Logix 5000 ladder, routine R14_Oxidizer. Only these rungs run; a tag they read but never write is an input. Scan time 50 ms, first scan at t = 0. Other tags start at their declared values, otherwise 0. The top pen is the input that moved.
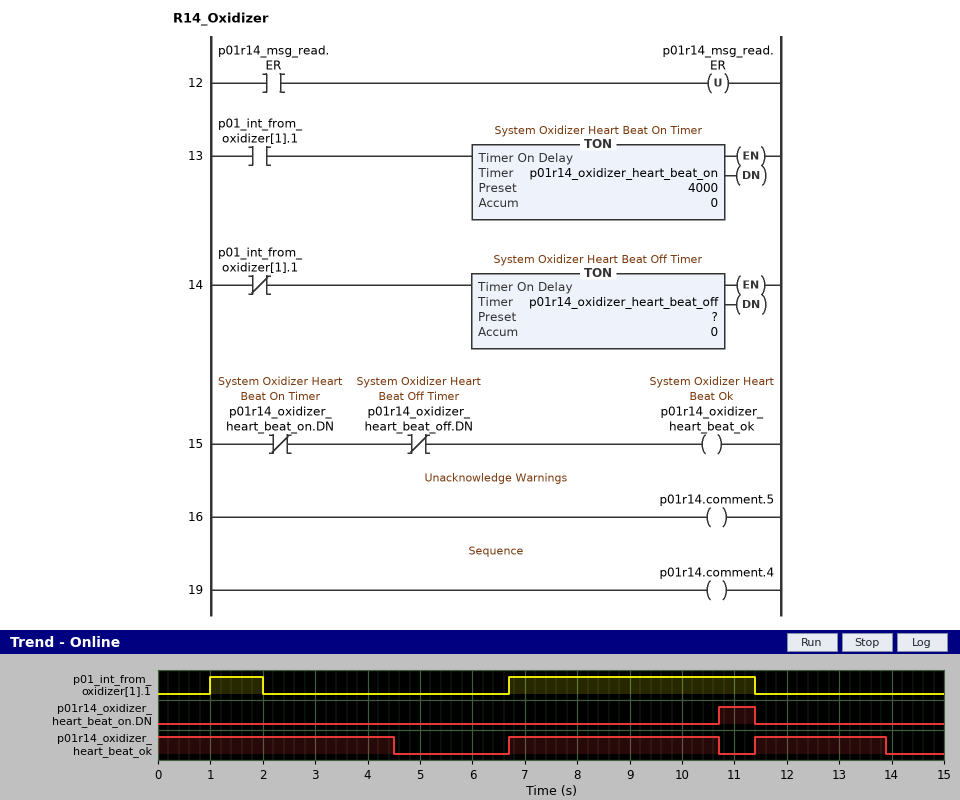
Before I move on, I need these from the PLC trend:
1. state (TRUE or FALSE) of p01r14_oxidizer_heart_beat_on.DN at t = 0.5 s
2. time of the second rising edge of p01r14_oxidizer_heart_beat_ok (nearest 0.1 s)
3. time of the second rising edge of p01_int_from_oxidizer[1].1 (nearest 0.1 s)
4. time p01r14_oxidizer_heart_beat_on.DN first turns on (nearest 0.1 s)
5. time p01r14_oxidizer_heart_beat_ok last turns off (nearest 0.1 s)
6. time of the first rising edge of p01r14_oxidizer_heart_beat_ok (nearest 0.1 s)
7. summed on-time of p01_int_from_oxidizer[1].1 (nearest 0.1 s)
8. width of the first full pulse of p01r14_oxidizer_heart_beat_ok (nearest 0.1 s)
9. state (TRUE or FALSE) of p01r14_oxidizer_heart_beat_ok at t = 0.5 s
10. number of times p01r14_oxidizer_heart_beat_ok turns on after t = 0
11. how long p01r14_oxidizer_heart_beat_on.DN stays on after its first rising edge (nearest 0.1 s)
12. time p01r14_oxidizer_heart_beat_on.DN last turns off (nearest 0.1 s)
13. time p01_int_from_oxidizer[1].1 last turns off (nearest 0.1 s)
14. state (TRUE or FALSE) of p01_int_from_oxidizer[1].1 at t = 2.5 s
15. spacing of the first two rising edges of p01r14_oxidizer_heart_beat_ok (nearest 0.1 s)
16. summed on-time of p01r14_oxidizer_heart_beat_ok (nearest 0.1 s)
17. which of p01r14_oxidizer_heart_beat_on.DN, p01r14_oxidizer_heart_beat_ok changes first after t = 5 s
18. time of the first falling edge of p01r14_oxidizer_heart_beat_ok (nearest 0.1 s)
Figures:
FALSE
11.4 s
6.7 s
10.7 s
13.9 s
6.7 s
5.7 s
4.0 s
TRUE
2
0.7 s
11.4 s
11.4 s
FALSE
4.7 s
11.0 s
p01r14_oxidizer_heart_beat_ok
4.5 s
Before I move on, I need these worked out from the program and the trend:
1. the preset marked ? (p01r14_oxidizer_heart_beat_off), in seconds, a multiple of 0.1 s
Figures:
2.5 s
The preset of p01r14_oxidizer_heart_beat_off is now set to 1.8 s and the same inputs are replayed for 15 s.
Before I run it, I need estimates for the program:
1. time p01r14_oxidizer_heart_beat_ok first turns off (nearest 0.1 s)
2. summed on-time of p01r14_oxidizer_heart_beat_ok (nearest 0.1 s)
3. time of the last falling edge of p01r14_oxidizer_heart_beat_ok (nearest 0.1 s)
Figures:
3.8 s
9.6 s
13.2 s
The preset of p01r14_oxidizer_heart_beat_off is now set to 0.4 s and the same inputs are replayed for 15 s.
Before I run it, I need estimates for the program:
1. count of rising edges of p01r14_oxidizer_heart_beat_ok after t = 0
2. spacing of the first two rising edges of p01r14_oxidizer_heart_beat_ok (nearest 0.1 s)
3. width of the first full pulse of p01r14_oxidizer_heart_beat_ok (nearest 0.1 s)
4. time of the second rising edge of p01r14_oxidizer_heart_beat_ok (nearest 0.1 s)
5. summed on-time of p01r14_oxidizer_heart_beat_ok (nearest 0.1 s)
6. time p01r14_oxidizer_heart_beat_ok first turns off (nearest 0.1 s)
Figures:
3
5.7 s
1.4 s
6.7 s
6.2 s
0.4 s
